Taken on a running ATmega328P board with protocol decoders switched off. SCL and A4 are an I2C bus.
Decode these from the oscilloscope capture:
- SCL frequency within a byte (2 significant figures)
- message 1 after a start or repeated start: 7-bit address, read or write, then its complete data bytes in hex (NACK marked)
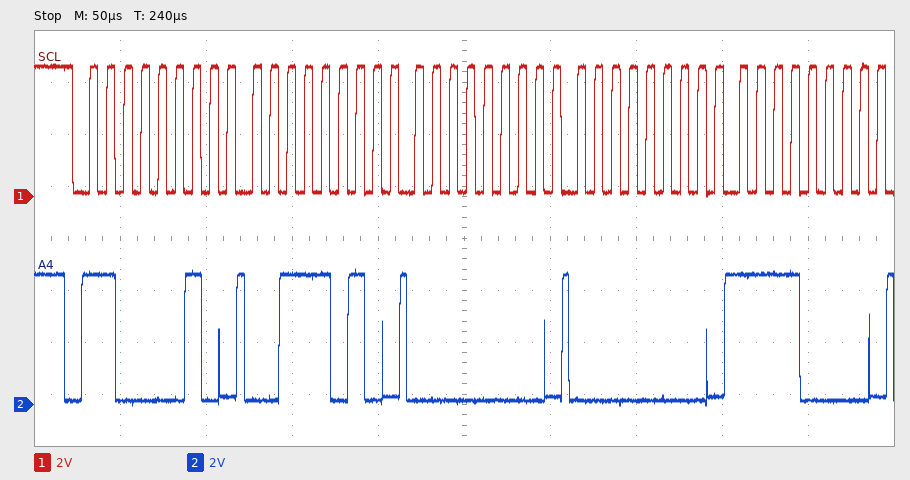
100 kHz
0x61 write: 3A 00 00 F0
